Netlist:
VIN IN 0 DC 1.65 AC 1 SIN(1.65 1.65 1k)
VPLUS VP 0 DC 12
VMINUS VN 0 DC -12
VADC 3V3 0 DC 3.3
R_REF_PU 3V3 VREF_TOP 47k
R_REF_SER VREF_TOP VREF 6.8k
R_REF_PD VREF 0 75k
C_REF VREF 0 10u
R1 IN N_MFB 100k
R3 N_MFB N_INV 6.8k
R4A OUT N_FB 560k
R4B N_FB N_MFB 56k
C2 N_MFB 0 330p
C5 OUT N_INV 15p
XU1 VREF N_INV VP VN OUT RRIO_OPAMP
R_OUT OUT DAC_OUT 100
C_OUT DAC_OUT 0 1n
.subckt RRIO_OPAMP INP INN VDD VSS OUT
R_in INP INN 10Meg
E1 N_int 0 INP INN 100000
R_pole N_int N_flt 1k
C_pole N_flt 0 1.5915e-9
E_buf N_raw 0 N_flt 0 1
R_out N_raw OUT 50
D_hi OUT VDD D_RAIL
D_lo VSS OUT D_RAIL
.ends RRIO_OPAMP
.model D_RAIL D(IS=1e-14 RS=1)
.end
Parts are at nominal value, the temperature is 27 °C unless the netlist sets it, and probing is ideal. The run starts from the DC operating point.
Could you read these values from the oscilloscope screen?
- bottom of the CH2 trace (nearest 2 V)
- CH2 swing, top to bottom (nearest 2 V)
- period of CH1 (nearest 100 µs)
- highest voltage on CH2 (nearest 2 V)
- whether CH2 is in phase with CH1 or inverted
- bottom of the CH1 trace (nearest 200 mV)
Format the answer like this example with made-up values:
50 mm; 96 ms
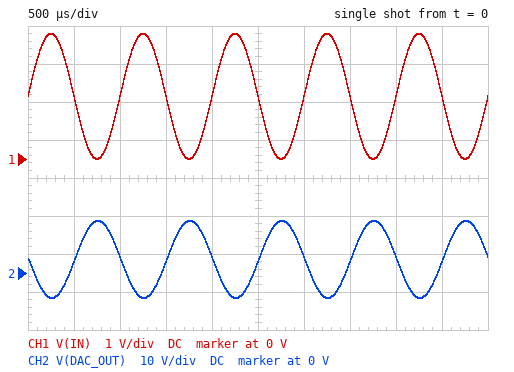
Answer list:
-6 V; 20 V; 1.0 ms; 14 V; inverted; 0 V
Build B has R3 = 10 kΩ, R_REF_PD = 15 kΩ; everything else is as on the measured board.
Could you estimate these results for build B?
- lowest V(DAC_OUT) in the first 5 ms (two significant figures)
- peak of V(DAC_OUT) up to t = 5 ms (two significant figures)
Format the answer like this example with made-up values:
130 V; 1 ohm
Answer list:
-15 V; 5.1 V
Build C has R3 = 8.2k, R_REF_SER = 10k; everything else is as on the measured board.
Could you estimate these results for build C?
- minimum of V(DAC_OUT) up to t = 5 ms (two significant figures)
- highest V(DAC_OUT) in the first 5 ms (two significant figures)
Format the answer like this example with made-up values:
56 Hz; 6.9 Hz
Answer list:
-6.9 V; 13 V
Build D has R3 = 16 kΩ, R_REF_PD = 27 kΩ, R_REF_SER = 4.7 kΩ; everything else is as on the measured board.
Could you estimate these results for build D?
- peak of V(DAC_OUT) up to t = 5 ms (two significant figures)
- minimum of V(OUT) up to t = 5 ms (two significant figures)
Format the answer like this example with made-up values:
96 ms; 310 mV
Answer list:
8.1 V; -12 V
